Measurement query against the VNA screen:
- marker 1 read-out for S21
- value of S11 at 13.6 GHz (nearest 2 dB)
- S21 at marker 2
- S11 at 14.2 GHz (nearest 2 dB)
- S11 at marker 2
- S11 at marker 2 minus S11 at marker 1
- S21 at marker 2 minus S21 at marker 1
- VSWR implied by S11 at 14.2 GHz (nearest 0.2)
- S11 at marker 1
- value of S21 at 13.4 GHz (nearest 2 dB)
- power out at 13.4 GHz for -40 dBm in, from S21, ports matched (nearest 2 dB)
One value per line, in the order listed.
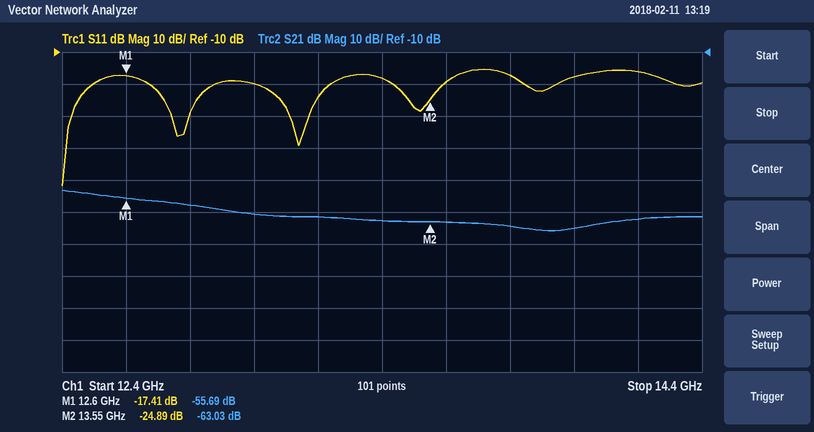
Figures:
-55.69 dB
-20 dB
-63.03 dB
-16 dB
-24.89 dB
-7.48 dB
-7.34 dB
1.4
-17.41 dB
-62 dB
-102 dBm
